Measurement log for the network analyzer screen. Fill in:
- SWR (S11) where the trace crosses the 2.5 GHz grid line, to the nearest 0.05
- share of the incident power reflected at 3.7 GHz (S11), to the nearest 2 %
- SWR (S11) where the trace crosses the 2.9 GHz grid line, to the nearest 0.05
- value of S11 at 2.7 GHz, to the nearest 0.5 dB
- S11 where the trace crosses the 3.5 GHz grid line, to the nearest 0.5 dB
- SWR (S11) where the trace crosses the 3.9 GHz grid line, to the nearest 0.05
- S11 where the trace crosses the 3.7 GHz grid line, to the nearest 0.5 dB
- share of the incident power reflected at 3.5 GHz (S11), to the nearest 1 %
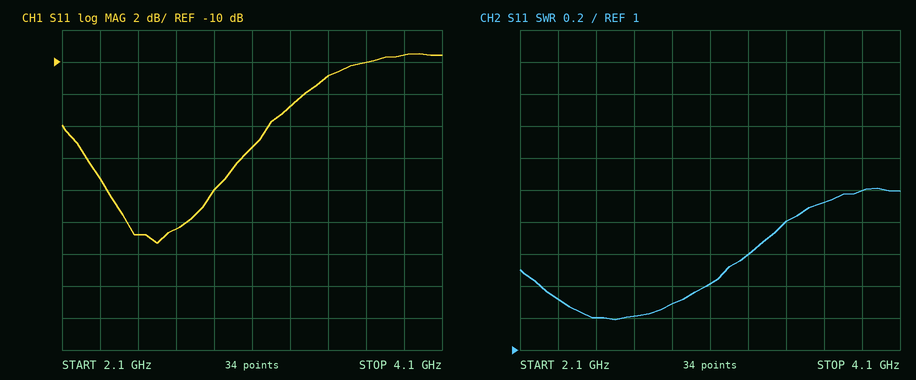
1.20
10 %
1.30
-20.5 dB
-11.0 dB
2.00
-10.0 dB
8 %
